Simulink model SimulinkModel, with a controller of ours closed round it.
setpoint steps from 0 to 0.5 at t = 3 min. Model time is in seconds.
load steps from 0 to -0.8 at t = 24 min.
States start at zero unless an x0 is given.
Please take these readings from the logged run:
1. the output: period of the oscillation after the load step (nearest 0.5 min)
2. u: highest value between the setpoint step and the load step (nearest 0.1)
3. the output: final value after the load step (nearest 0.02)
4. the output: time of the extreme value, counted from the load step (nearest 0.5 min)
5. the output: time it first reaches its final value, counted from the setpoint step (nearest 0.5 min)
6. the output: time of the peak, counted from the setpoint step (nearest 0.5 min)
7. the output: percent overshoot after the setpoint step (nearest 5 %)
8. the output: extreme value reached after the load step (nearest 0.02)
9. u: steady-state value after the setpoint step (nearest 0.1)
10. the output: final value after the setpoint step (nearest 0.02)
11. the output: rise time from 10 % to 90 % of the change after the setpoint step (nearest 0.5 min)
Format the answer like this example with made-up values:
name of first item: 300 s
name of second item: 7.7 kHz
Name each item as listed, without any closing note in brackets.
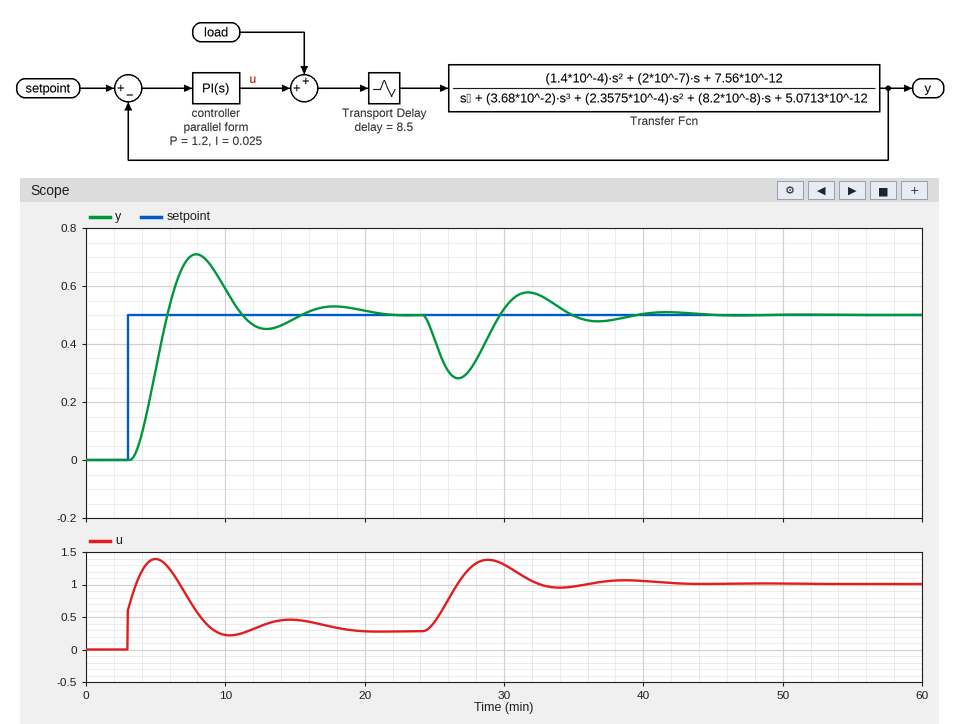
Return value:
the output: period of the oscillation after the load step: 10.0 min
u: highest value between the setpoint step and the load step: 1.4
the output: final value after the load step: 0.50
the output: time of the extreme value, counted from the load step: 2.5 min
the output: time it first reaches its final value, counted from the setpoint step: 3.0 min
the output: time of the peak, counted from the setpoint step: 5.0 min
the output: percent overshoot after the setpoint step: 40 %
the output: extreme value reached after the load step: 0.28
u: steady-state value after the setpoint step: 0.3
the output: final value after the setpoint step: 0.50
the output: rise time from 10 % to 90 % of the change after the setpoint step: 2.0 min
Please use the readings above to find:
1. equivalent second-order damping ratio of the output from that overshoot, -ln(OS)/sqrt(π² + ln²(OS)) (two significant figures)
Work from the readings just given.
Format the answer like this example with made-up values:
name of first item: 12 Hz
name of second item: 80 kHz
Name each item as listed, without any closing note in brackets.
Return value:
equivalent second-order damping ratio of the output from that overshoot, -ln(OS)/sqrt(π² + ln²(OS)): 0.28
